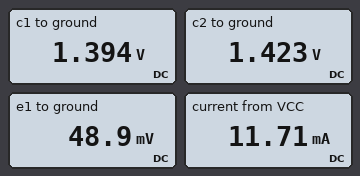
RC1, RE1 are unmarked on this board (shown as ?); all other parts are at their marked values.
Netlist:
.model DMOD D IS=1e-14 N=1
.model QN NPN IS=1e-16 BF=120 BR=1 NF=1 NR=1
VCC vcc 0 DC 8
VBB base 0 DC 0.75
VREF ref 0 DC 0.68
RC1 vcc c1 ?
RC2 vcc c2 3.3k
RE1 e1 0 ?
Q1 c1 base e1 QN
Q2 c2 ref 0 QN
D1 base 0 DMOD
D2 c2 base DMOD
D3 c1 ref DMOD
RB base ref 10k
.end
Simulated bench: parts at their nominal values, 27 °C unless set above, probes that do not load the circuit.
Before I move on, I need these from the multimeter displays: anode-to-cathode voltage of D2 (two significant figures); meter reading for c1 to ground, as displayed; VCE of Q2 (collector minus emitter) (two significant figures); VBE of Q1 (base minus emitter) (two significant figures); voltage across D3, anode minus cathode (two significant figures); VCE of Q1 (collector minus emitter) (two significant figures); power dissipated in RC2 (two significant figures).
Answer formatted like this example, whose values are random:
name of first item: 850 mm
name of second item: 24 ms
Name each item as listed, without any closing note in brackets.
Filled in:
anode-to-cathode voltage of D2: 670 mV
meter reading for c1 to ground, as displayed: 1.394 V
VCE of Q2 (collector minus emitter): 1.4 V
VBE of Q1 (base minus emitter): 700 mV
voltage across D3, anode minus cathode: 710 mV
VCE of Q1 (collector minus emitter): 1.3 V
power dissipated in RC2: 13 mW
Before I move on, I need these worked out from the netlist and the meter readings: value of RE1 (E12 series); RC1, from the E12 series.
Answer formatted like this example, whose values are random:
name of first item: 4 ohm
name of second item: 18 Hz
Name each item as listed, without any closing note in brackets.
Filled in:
value of RE1: 820 Ω
RC1, from the E12 series: 680 Ω
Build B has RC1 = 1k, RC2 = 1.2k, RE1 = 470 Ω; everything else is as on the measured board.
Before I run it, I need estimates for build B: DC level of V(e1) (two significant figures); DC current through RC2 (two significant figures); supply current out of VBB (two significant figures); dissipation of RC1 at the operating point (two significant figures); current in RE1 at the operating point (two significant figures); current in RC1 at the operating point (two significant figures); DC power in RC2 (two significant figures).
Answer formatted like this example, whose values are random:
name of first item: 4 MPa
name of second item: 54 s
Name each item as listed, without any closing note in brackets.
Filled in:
DC level of V(e1): 40 mV
DC current through RC2: 5.5 mA
supply current out of VBB: 34 mA
dissipation of RC1 at the operating point: 44 mW
current in RE1 at the operating point: 85 µA
current in RC1 at the operating point: 6.6 mA
DC power in RC2: 36 mW
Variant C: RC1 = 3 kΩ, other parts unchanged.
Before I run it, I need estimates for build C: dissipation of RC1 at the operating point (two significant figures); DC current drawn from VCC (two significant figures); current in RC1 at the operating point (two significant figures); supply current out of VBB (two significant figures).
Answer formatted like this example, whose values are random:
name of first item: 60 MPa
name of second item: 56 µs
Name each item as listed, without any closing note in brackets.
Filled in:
dissipation of RC1 at the operating point: 15 mW
DC current drawn from VCC: 4.2 mA
current in RC1 at the operating point: 2.2 mA
supply current out of VBB: 37 mA
